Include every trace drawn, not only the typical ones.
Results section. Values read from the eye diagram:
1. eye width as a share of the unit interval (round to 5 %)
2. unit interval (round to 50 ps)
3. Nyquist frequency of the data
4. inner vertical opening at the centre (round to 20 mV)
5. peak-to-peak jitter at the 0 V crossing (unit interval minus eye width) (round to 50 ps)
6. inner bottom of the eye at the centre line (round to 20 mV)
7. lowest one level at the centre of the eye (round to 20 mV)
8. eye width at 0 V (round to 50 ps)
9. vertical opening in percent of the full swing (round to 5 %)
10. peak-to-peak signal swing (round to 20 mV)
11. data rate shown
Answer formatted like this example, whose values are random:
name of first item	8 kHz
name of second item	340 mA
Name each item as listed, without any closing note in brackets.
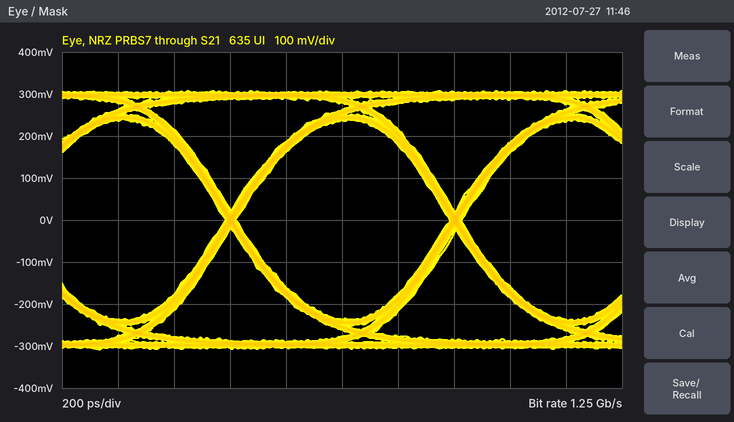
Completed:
eye width as a share of the unit interval	95 %
unit interval	800 ps
Nyquist frequency of the data	625 MHz
inner vertical opening at the centre	480 mV
peak-to-peak jitter at the 0 V crossing (unit interval minus eye width)	50 ps
inner bottom of the eye at the centre line	-240 mV
lowest one level at the centre of the eye	240 mV
eye width at 0 V	750 ps
vertical opening in percent of the full swing	75 %
peak-to-peak signal swing	620 mV
data rate shown	1.25 Gb/s
